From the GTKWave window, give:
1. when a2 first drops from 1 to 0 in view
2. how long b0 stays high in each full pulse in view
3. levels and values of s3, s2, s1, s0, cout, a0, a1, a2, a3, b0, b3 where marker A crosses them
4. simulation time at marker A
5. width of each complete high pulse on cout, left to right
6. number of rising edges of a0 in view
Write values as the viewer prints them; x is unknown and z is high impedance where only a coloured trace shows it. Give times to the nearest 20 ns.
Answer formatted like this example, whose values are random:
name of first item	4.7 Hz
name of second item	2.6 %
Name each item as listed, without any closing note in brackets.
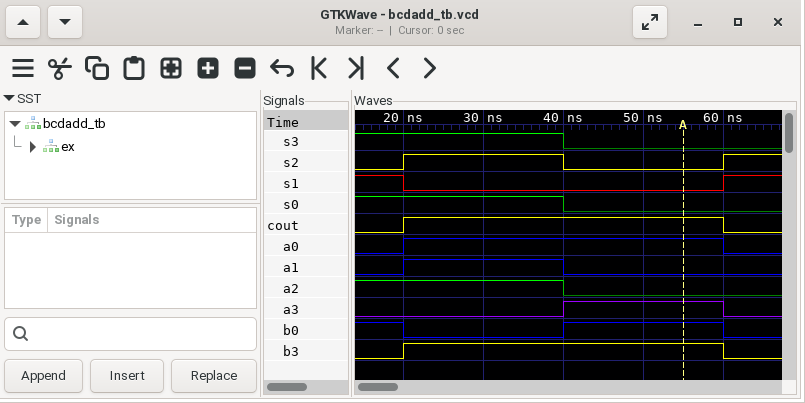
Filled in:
when a2 first drops from 1 to 0 in view	40 ns
how long b0 stays high in each full pulse in view	20 ns
levels and values of s3, s2, s1, s0, cout, a0, a1, a2, a3, b0, b3 where marker A crosses them	s3=0, s2=0, s1=0, s0=0, cout=1, a0=1, a1=0, a2=0, a3=1, b0=1, b3=1
simulation time at marker A	60 ns
width of each complete high pulse on cout, left to right	40 ns
number of rising edges of a0 in view	1
